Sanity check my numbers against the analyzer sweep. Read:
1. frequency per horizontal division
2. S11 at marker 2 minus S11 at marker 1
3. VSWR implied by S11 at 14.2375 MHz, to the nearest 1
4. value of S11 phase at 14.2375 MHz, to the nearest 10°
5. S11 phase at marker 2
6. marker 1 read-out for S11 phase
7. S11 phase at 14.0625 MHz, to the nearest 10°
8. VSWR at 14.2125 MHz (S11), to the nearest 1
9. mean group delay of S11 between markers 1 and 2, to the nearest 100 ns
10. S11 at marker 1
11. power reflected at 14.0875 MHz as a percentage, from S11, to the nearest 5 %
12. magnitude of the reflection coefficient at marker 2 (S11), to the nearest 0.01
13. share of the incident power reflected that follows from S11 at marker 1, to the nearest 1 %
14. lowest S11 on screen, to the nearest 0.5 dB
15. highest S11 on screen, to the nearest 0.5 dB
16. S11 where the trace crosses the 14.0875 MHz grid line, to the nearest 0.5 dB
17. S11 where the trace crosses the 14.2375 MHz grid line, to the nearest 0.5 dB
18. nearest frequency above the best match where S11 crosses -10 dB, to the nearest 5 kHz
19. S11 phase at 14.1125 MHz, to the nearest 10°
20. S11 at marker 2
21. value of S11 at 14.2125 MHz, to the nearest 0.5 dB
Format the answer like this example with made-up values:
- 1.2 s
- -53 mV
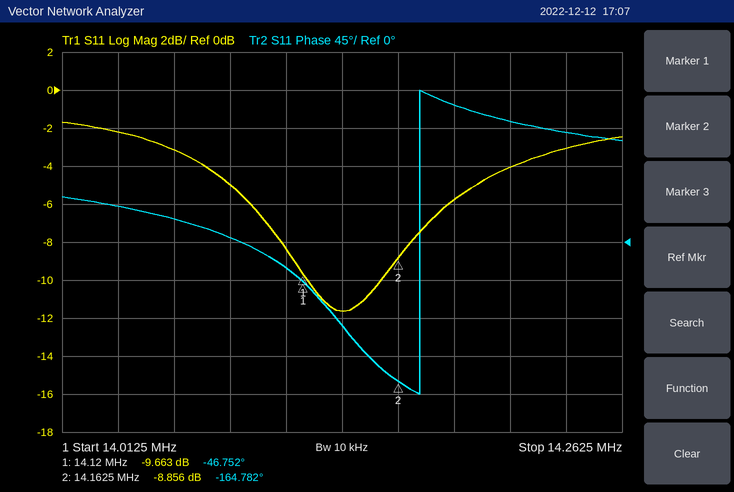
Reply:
- 25 kHz
- 0.807 dB
- 6
- 130°
- -164.782°
- -46.752°
- 30°
- 4
- 7.7 µs
- -9.663 dB
- 30 %
- 0.36
- 11 %
- -11.5 dB
- -1.5 dB
- -5.0 dB
- -3.0 dB
- 14.155 MHz
- -30°
- -8.856 dB
- -4.0 dB
